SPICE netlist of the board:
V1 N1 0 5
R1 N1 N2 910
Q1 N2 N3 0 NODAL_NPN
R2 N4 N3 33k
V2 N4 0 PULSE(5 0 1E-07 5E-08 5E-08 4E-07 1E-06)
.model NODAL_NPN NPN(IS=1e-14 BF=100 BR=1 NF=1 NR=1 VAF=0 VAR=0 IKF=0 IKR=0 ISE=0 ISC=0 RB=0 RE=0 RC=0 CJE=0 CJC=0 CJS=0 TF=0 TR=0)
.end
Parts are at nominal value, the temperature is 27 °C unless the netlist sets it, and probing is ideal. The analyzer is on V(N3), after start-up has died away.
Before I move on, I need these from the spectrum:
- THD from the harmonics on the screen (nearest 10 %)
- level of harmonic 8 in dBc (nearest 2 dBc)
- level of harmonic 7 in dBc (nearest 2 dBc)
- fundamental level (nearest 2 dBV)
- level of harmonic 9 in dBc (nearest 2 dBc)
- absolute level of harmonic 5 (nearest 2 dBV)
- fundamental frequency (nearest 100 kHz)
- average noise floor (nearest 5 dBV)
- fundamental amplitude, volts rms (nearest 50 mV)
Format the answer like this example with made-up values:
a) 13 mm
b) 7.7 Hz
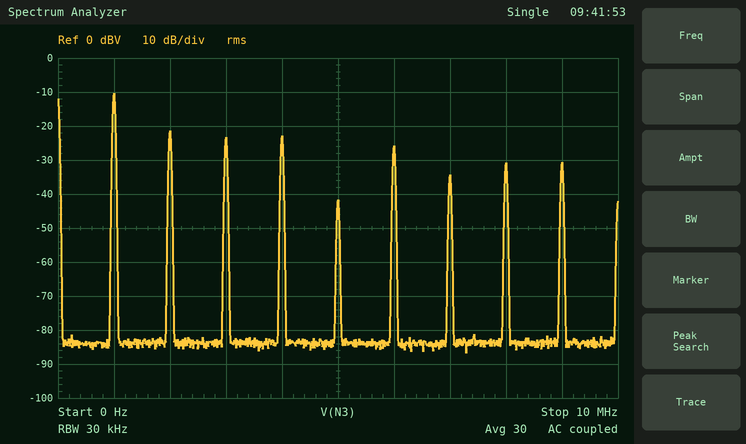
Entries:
a) 50 %
b) -20 dBc
c) -24 dBc
d) -10 dBV
e) -20 dBc
f) -42 dBV
g) 1.0 MHz
h) -85 dBV
i) 300 mV
